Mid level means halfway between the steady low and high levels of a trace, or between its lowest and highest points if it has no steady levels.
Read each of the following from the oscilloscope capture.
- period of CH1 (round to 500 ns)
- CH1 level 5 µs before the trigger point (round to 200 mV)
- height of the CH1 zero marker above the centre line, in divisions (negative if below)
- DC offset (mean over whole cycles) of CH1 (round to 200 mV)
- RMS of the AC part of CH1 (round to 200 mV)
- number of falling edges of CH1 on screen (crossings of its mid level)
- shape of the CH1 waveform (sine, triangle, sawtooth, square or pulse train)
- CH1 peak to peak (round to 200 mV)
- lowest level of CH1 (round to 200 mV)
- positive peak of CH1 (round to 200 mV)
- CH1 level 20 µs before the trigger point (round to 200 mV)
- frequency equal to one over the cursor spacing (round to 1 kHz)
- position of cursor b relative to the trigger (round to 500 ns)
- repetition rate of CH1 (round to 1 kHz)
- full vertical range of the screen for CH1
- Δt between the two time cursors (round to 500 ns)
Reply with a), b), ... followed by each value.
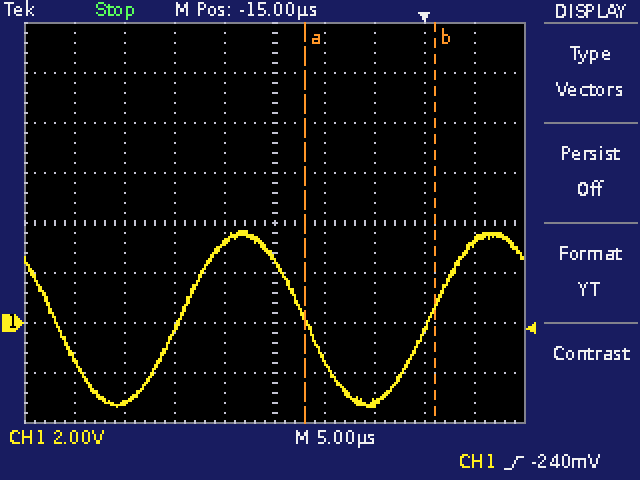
a) 25.0 µs
b) -3.2 V
c) -2.0 div
d) 200 mV
e) 2.4 V
f) 2
g) sine
h) 7.0 V
i) -3.4 V
j) 3.6 V
k) 3.2 V
l) 77 kHz
m) +1.0 µs
n) 40 kHz
o) 16 V
p) 13.0 µs
